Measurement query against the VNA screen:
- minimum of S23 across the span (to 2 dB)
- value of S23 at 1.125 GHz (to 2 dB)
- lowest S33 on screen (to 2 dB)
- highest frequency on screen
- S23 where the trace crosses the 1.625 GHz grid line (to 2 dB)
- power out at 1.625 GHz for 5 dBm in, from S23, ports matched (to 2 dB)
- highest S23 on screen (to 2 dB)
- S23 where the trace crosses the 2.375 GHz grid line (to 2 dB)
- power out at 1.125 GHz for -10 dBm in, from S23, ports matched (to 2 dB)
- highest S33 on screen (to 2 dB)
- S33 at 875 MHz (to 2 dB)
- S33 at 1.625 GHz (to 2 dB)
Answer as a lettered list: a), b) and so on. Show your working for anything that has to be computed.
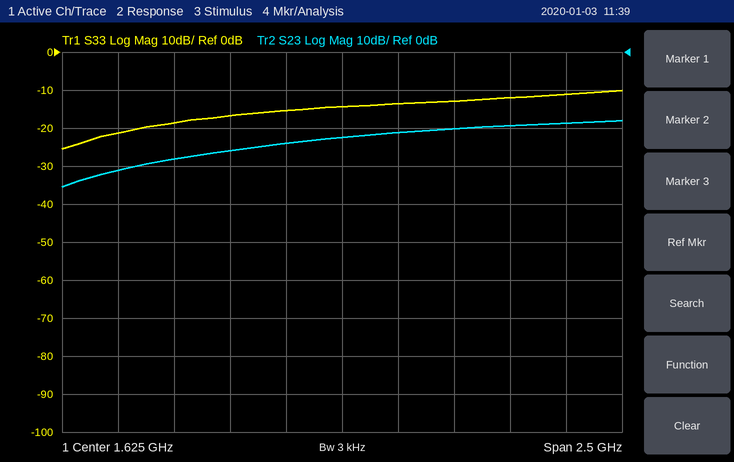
a) -36 dB
b) -26 dB
c) -26 dB
d) 2.875 GHz
e) -22 dB
f) 5 dBm + (-22 dB) = -18 dBm
g) -18 dB
h) -20 dB
i) -10 dBm + (-26 dB) = -36 dBm
j) -10 dB
k) -18 dB
l) -14 dB
